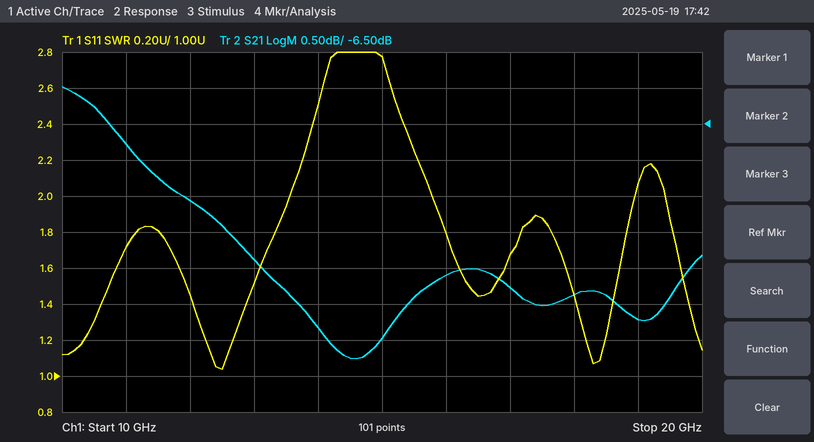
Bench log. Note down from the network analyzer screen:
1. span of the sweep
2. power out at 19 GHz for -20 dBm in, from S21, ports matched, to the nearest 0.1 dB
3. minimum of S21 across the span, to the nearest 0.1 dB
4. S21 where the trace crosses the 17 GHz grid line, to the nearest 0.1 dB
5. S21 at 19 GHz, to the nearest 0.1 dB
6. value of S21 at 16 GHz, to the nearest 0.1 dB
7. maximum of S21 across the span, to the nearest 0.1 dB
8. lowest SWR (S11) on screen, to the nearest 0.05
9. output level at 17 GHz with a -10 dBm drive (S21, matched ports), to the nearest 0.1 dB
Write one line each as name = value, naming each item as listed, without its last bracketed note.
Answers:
span of the sweep = 10 GHz
power out at 19 GHz for -20 dBm in, from S21, ports matched, to the nearest 0.1 dB = -29.2 dBm
minimum of S21 across the span, to the nearest 0.1 dB = -9.8 dB
S21 where the trace crosses the 17 GHz grid line, to the nearest 0.1 dB = -8.8 dB
S21 at 19 GHz, to the nearest 0.1 dB = -9.2 dB
value of S21 at 16 GHz, to the nearest 0.1 dB = -8.6 dB
maximum of S21 across the span, to the nearest 0.1 dB = -6.0 dB
lowest SWR (S11) on screen, to the nearest 0.05 = 1.05
output level at 17 GHz with a -10 dBm drive (S21, matched ports), to the nearest 0.1 dB = -18.8 dBm
